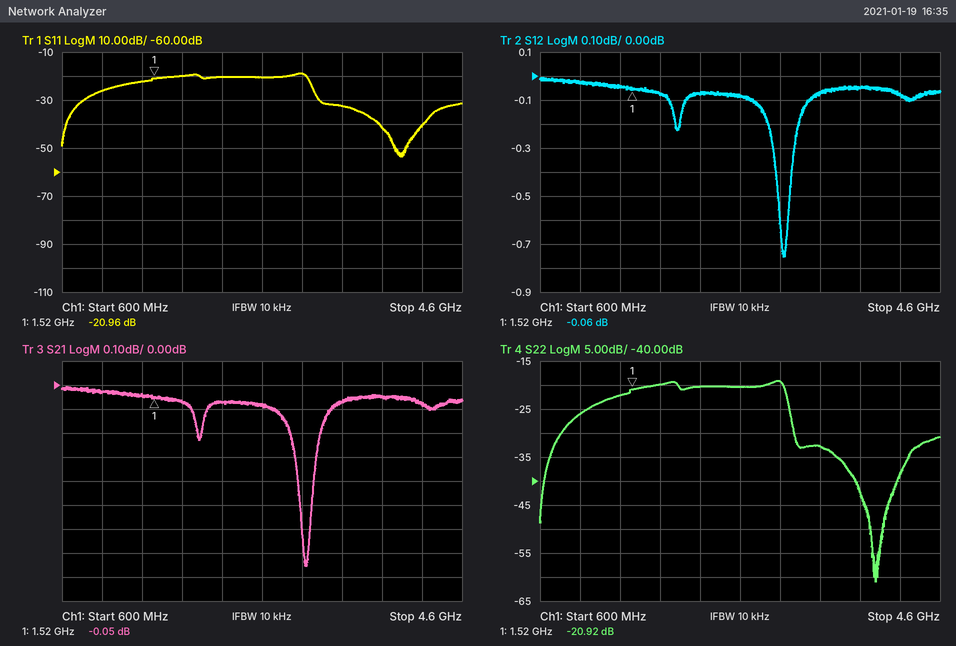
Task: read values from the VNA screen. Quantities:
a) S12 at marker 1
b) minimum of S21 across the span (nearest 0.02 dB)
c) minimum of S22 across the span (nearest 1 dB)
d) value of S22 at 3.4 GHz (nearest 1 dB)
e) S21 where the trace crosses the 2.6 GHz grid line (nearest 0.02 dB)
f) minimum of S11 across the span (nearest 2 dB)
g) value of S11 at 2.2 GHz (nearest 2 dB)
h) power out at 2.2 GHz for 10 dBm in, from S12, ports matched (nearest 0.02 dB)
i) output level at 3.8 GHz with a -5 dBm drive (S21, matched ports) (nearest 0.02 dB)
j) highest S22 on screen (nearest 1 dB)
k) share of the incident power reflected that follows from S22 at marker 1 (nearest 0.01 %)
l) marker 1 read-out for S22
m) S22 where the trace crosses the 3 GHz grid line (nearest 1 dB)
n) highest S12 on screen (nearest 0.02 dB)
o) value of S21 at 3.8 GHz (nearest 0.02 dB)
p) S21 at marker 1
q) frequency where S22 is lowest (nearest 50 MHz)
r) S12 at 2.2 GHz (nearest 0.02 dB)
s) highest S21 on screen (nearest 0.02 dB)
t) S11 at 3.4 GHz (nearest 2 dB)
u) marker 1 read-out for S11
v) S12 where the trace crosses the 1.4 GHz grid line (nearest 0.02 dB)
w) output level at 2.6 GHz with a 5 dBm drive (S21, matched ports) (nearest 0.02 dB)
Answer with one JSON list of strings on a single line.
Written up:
["-0.06 dB", "-0.76 dB", "-61 dB", "-33 dB", "-0.08 dB", "-54 dB", "-20 dB", "9.92 dBm", "-5.04 dBm", "-19 dB", "0.81 %", "-20.92 dB", "-19 dB", "0.00 dB", "-0.04 dB", "-0.05 dB", "3.95 GHz", "-0.08 dB", "0.00 dB", "-32 dB", "-20.96 dB", "-0.04 dB", "4.92 dBm"]
